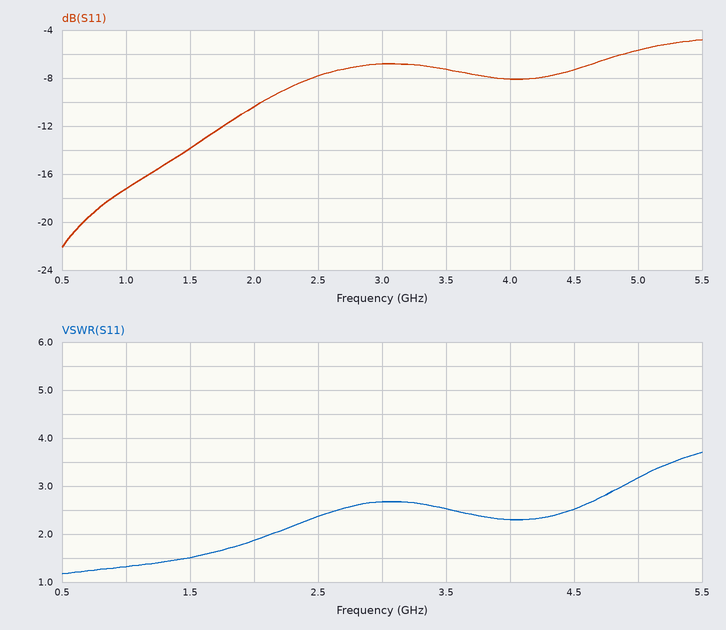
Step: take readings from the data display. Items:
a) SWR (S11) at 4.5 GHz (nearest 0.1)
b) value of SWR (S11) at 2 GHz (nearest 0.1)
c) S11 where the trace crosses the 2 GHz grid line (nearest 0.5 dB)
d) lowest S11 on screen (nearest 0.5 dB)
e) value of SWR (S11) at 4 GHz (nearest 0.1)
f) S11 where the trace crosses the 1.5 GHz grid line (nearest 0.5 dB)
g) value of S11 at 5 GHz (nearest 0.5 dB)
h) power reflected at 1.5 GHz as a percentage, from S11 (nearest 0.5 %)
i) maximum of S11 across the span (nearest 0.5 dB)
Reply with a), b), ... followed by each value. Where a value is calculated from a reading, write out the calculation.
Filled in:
a) 2.5
b) 1.9
c) -10.5 dB
d) -22.0 dB
e) 2.3
f) -14.0 dB
g) -5.5 dB
h) 10^(-14/10) ≈ 4.0 %
i) -5.0 dB
